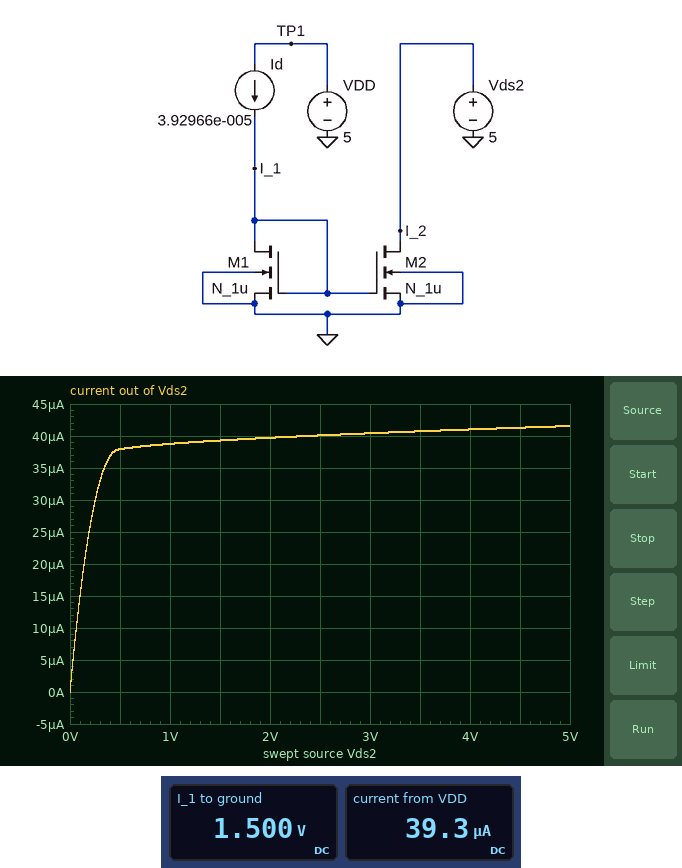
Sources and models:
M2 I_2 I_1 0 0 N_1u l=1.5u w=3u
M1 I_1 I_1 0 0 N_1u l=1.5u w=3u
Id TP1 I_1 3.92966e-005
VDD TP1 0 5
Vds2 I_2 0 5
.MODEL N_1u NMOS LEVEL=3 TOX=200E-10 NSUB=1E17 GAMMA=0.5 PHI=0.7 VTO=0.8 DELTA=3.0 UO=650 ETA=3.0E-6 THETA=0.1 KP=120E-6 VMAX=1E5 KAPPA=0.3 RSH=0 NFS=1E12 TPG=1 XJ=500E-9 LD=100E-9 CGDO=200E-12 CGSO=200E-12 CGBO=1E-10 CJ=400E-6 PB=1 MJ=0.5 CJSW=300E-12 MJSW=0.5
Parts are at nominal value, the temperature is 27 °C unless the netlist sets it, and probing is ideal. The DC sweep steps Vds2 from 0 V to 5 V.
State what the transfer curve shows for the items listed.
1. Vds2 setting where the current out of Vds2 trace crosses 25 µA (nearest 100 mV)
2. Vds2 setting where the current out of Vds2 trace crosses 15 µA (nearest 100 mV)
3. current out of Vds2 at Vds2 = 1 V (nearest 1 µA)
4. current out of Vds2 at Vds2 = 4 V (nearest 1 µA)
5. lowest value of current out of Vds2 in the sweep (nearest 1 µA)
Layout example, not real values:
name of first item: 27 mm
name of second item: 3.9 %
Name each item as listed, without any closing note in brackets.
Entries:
Vds2 setting where the current out of Vds2 trace crosses 25 µA: 200 mV
Vds2 setting where the current out of Vds2 trace crosses 15 µA: 100 mV
current out of Vds2 at Vds2 = 1 V: 39 µA
current out of Vds2 at Vds2 = 4 V: 41 µA
lowest value of current out of Vds2 in the sweep: 0 A
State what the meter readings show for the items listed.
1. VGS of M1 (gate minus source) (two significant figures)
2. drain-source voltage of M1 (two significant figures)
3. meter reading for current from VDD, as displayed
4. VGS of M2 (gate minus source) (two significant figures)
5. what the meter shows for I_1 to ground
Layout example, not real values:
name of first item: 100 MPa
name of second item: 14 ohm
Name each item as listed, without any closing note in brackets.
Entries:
VGS of M1 (gate minus source): 1.5 V
drain-source voltage of M1: 1.5 V
meter reading for current from VDD, as displayed: 39.3 µA
VGS of M2 (gate minus source): 1.5 V
what the meter shows for I_1 to ground: 1.500 V
